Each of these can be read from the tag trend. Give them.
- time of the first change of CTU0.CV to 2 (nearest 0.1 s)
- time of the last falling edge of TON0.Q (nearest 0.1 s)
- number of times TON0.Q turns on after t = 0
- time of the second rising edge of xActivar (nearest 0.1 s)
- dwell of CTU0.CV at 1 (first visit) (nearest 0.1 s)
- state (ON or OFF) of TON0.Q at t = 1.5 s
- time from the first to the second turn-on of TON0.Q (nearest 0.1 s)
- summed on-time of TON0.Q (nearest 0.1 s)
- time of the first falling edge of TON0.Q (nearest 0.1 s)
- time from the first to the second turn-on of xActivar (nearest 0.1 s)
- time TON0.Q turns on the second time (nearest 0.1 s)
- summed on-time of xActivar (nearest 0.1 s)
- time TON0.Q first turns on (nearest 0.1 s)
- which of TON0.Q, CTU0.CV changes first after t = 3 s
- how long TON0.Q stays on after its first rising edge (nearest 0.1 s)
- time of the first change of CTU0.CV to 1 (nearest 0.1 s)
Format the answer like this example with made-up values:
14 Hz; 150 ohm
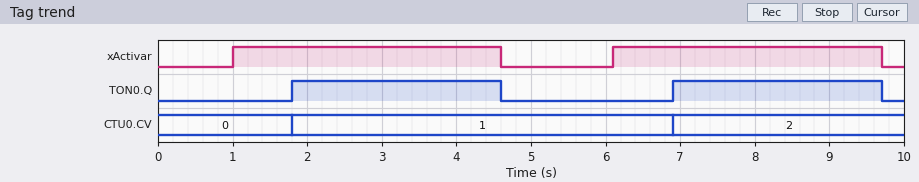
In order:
6.9 s; 9.7 s; 2; 6.1 s; 5.1 s; OFF; 5.1 s; 5.6 s; 4.6 s; 5.1 s; 6.9 s; 7.2 s; 1.8 s; TON0.Q; 2.8 s; 1.8 s
